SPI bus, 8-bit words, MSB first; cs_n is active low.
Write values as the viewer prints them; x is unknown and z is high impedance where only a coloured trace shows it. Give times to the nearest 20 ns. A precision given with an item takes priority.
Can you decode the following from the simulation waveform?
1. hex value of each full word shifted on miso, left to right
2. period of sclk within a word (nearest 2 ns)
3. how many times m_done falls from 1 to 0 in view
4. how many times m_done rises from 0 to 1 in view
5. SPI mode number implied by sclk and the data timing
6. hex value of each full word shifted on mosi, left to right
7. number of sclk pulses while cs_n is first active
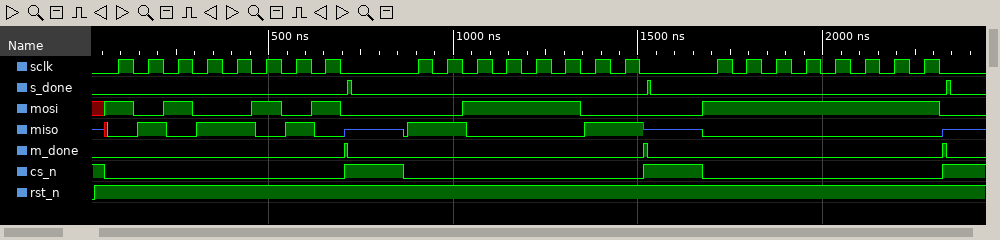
5A, C3, 00
80 ns
3
3
0
A5, 3C, FF
8
